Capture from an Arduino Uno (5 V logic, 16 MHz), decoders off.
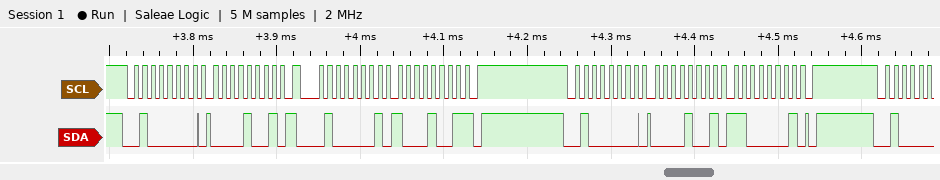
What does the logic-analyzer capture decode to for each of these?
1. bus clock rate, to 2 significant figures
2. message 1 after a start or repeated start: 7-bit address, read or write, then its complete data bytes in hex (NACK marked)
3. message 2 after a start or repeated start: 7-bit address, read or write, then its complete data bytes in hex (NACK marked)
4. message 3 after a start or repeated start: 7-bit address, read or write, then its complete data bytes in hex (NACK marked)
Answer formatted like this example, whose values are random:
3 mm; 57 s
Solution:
100 kHz; 0x20 write: 09; 0x20 read: 89 NACK; 0x20 write: 09 C1
